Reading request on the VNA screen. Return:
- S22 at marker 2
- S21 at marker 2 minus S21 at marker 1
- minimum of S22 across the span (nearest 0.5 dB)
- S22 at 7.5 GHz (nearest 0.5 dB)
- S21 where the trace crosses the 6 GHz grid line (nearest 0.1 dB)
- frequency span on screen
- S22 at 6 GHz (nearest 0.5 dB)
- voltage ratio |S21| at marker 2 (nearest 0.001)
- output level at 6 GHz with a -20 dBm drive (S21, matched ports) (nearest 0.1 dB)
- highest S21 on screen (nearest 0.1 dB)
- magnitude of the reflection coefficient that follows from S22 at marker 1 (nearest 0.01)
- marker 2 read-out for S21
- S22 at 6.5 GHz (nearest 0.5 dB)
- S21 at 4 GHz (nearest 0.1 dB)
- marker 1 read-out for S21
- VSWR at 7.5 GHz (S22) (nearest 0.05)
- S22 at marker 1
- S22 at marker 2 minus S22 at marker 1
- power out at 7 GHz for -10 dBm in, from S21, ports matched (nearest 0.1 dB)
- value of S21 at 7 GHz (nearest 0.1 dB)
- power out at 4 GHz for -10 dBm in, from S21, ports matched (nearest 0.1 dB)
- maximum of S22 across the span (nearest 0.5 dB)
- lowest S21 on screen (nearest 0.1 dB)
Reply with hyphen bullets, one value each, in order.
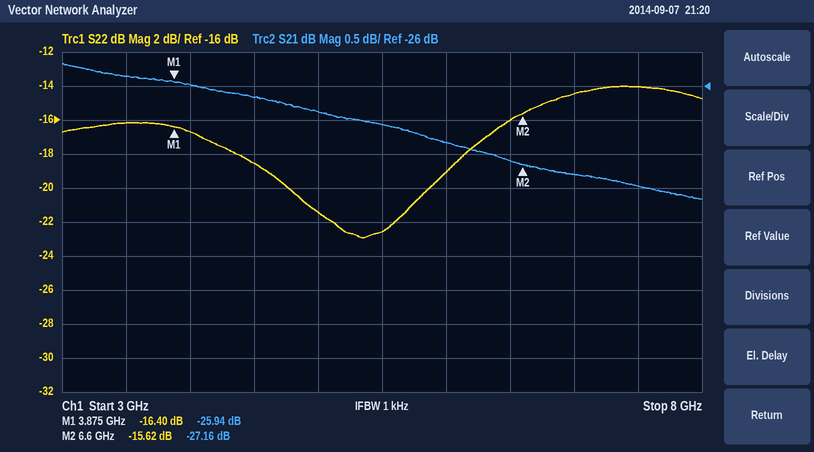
- -15.62 dB
- -1.22 dB
- -23.0 dB
- -14.0 dB
- -26.8 dB
- 5 GHz
- -19.0 dB
- 0.044
- -46.8 dBm
- -25.7 dB
- 0.15
- -27.16 dB
- -16.0 dB
- -26.0 dB
- -25.94 dB
- 1.50
- -16.40 dB
- 0.78 dB
- -37.3 dBm
- -27.3 dB
- -36.0 dBm
- -14.0 dB
- -27.7 dB
